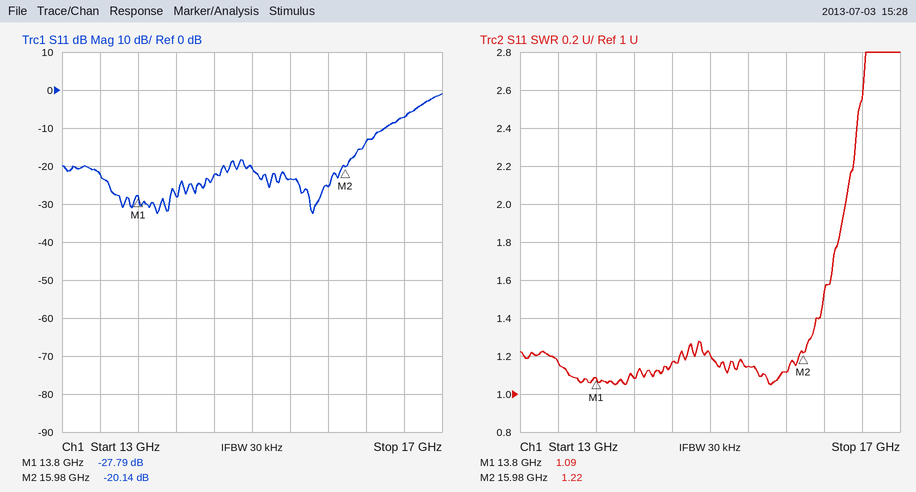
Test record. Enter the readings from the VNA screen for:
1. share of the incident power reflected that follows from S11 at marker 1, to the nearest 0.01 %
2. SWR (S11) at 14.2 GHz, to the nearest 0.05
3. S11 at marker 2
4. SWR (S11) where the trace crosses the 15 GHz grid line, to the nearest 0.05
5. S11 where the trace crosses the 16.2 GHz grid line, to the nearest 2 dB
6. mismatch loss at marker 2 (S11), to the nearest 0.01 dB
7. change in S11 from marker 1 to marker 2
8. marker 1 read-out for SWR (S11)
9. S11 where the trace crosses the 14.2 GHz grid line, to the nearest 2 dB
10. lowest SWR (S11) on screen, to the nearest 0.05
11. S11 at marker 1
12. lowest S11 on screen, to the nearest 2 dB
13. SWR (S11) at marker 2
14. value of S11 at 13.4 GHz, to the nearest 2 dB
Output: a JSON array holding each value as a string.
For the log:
["0.17 %", "1.10", "-20.14 dB", "1.20", "-14 dB", "0.04 dB", "7.65 dB", "1.09", "-28 dB", "1.05", "-27.79 dB", "-32 dB", "1.22", "-22 dB"]
